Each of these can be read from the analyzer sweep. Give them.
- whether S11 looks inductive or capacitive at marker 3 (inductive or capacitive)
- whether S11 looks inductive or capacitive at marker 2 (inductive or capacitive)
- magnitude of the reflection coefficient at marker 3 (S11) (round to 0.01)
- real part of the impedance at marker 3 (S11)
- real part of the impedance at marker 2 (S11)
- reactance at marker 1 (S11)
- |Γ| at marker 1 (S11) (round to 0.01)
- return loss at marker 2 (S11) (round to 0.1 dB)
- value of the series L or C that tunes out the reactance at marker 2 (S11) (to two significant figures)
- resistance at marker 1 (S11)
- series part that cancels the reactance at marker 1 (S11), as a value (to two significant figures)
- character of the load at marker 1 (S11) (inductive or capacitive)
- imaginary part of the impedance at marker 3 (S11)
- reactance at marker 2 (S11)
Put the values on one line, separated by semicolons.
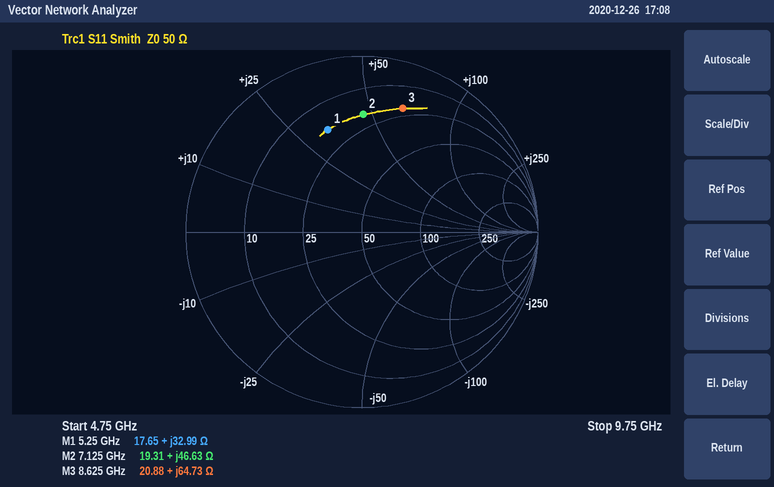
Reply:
inductive; inductive; 0.74; 20.88 Ω; 19.31 Ω; +32.99 Ω; 0.61; 3.5 dB; 480 fF; 17.65 Ω; 920 fF; inductive; +64.73 Ω; +46.63 Ω
